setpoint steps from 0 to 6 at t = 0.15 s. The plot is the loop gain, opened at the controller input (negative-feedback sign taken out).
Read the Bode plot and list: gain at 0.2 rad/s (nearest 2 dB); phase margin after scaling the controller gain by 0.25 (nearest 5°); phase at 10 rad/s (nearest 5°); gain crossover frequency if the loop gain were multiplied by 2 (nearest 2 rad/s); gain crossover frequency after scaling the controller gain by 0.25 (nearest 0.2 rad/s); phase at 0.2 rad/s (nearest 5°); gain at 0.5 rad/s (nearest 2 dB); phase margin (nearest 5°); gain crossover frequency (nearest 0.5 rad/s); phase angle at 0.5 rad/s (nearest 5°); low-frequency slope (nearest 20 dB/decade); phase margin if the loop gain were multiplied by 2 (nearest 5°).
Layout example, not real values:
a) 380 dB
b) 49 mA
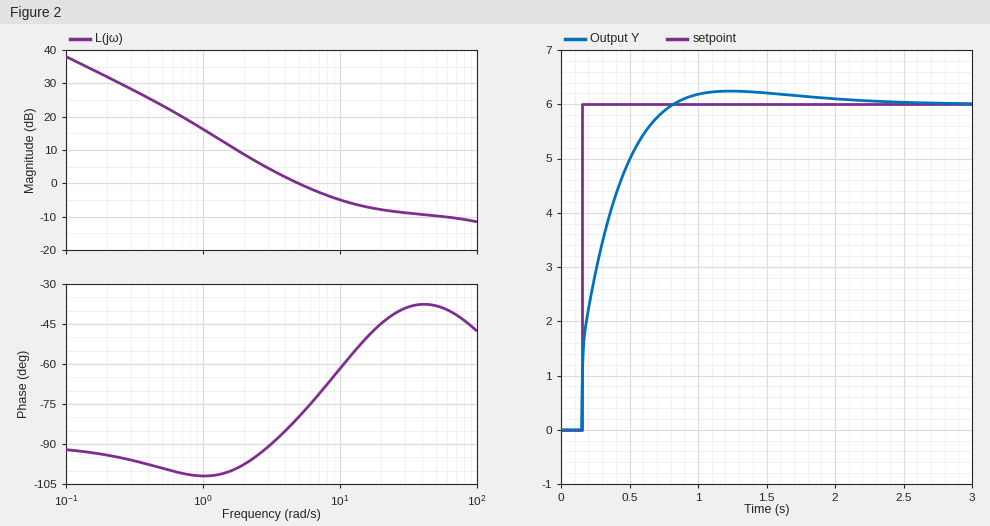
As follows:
a) 32 dB
b) 80°
c) -60°
d) 12 rad/s
e) 1.4 rad/s
f) -95°
g) 24 dB
h) 100°
i) 5.0 rad/s
j) -100°
k) -20 dB/decade
l) 125°
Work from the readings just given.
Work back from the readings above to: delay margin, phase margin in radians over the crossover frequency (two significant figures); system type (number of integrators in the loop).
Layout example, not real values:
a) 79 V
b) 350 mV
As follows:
a) 0.35 s
b) 1
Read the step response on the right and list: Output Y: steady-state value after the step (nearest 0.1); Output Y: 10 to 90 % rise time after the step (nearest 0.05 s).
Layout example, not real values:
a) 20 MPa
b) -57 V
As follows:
a) 6.0
b) 0.45 s
